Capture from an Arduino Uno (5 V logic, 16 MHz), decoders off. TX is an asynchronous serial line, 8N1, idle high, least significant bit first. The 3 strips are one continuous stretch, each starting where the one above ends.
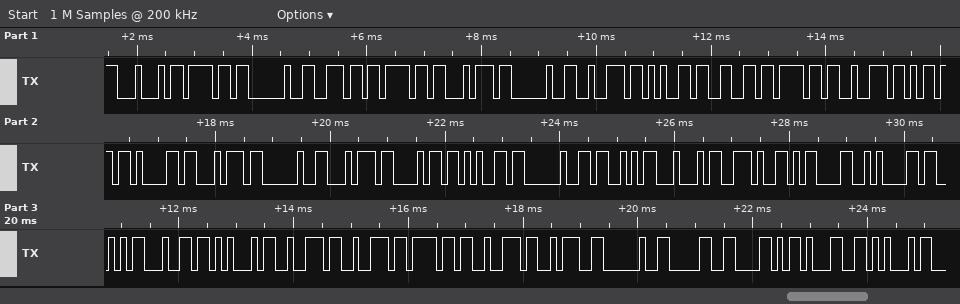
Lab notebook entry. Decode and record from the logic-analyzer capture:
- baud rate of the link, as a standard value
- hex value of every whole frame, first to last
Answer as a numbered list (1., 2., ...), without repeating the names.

1. 9600 baud
2. 44 6F 20 6E 6F 74 20 72 65 66 6F 72 6D 61 74 20 74 68 65 20 53 44 2E 0D 0A 53 64 45 72 72 6F 72 3A 20 30 58 31 45
